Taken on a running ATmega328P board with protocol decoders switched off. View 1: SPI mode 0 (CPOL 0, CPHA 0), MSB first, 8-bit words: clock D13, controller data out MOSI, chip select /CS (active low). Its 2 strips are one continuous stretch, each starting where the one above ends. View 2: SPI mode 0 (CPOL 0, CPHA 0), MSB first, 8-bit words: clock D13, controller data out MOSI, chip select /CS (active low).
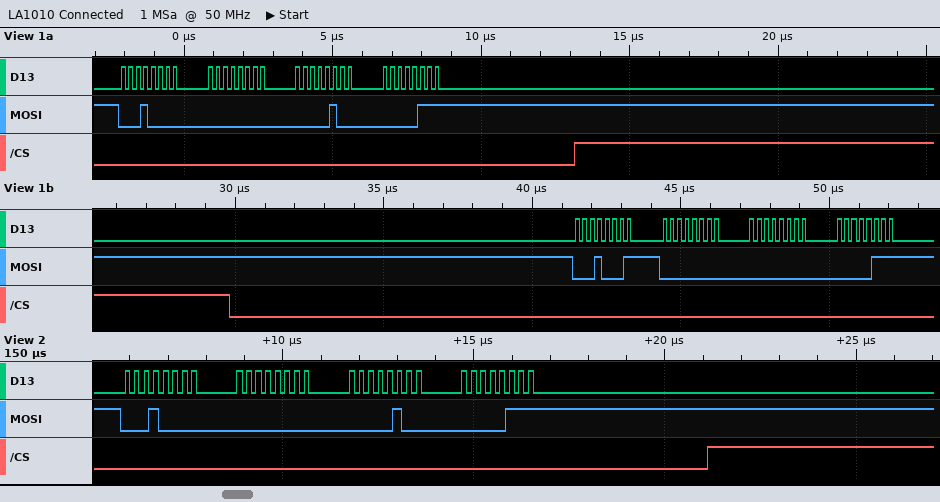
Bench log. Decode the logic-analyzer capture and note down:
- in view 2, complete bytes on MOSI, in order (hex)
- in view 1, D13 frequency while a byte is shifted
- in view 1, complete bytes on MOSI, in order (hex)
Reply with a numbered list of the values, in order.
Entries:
1. 0x10 0x00 0x04 0x07
2. 4 MHz
3. 10 00 04 07 11 00 00 07
